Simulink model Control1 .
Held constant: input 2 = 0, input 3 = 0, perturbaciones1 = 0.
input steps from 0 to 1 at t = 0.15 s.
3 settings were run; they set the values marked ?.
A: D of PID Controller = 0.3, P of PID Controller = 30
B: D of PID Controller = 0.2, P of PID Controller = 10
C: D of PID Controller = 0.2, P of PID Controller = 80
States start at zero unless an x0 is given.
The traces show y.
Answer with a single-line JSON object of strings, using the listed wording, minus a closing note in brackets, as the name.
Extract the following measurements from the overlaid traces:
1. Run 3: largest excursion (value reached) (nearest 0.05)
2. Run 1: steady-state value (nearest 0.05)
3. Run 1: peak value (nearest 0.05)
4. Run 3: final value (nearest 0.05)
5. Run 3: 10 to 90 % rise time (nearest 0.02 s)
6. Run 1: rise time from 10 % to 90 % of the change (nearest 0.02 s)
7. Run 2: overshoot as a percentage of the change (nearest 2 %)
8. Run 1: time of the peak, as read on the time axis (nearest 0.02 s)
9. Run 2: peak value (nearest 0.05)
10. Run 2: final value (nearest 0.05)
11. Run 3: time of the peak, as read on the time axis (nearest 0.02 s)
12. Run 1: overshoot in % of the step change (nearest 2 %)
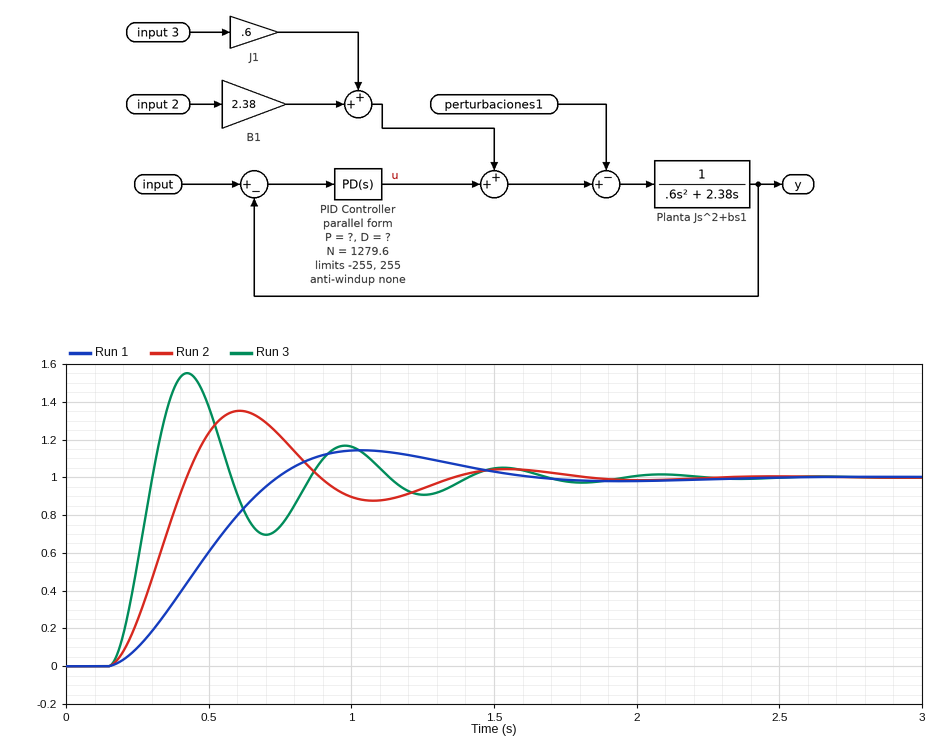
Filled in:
{"Run 3: largest excursion (value reached)": "1.55", "Run 1: steady-state value": "1.00", "Run 1: peak value": "1.15", "Run 3: final value": "1.00", "Run 3: 10 to 90 % rise time": "0.10 s", "Run 1: rise time from 10 % to 90 % of the change": "0.42 s", "Run 2: overshoot as a percentage of the change": "36 %", "Run 1: time of the peak, as read on the time axis": "1.04 s", "Run 2: peak value": "1.35", "Run 2: final value": "1.00", "Run 3: time of the peak, as read on the time axis": "0.42 s", "Run 1: overshoot in % of the step change": "14 %"}
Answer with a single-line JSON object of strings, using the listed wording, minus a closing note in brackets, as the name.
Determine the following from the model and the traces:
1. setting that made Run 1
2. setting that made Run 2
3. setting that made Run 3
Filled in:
{"setting that made Run 1": "B", "setting that made Run 2": "A", "setting that made Run 3": "C"}
